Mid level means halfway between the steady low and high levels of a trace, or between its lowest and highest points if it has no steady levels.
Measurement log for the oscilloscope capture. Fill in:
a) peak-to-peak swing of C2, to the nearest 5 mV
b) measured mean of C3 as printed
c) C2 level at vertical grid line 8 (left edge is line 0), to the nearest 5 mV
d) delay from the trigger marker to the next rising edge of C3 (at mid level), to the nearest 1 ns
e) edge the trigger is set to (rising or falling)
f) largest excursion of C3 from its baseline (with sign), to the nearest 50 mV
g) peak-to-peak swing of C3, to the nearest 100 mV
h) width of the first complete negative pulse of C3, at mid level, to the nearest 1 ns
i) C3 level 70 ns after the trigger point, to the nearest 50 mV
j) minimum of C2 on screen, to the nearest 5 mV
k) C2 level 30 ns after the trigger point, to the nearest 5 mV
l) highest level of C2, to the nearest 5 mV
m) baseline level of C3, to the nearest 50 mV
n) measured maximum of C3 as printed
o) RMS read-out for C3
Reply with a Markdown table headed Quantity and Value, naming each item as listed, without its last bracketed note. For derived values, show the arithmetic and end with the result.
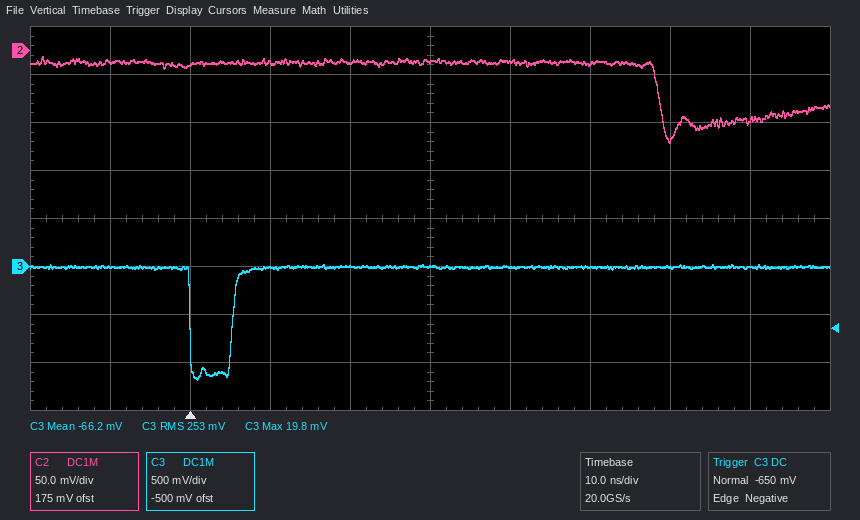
| Quantity | Value |
|---|---|
| peak-to-peak swing of C2, to the nearest 5 mV | -5 mV − (-95 mV) = 90 mV |
| measured mean of C3 as printed | -66.2 mV |
| C2 level at vertical grid line 8 (left edge is line 0), to the nearest 5 mV | -90 mV |
| delay from the trigger marker to the next rising edge of C3 (at mid level), to the nearest 1 ns | 5 ns |
| edge the trigger is set to | falling |
| largest excursion of C3 from its baseline (with sign), to the nearest 50 mV | -1.15 V |
| peak-to-peak swing of C3, to the nearest 100 mV | 1.20 V |
| width of the first complete negative pulse of C3, at mid level, to the nearest 1 ns | 5 ns |
| C3 level 70 ns after the trigger point, to the nearest 50 mV | 0 mV |
| minimum of C2 on screen, to the nearest 5 mV | -95 mV |
| C2 level 30 ns after the trigger point, to the nearest 5 mV | -10 mV |
| highest level of C2, to the nearest 5 mV | -5 mV |
| baseline level of C3, to the nearest 50 mV | 0 mV |
| measured maximum of C3 as printed | 19.8 mV |
| RMS read-out for C3 | 253 mV |
